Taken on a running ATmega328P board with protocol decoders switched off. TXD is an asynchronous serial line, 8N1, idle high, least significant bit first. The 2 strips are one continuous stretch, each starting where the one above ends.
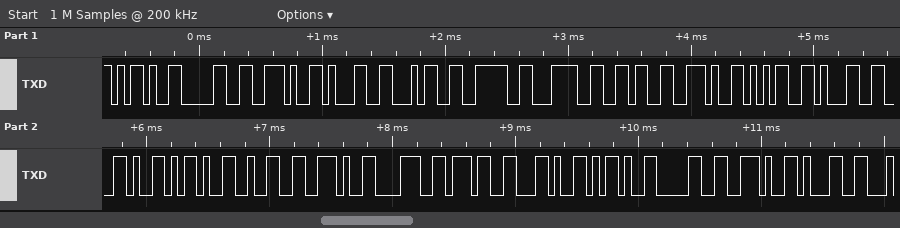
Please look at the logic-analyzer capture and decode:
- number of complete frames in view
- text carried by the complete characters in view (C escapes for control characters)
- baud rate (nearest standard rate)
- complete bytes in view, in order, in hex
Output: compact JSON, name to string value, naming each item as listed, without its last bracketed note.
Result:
{"number of complete frames in view": "22", "text carried by the complete characters in view": "\"-0.14><6.51,-2.87,-0.1\"", "baud rate": "19200 baud", "complete bytes in view, in order, in hex": "2D 30 2E 31 34 3E 3C 36 2E 35 31 2C 2D 32 2E 38 37 2C 2D 30 2E 31"}
